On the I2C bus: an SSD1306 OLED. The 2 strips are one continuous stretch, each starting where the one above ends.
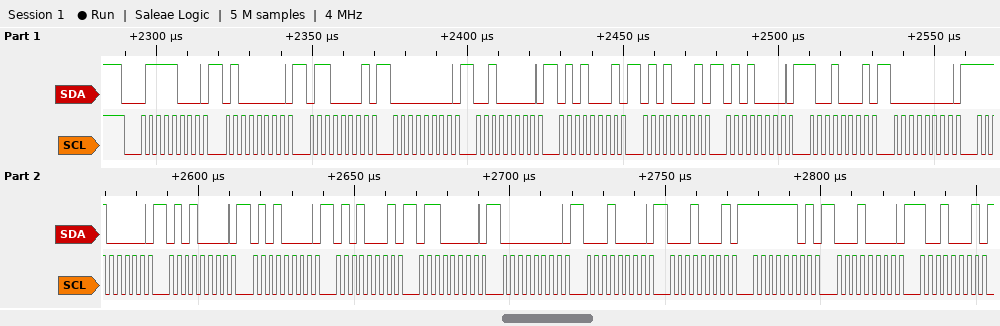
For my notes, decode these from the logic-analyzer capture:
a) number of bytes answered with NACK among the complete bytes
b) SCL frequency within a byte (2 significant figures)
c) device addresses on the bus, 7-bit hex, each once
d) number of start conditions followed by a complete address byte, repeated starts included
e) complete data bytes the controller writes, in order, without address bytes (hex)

0
400 kHz
0x3C
1
40 61 00 20 51 51 50 91 00 E0 50 50 51 60 00 10 11 FD 10 91
